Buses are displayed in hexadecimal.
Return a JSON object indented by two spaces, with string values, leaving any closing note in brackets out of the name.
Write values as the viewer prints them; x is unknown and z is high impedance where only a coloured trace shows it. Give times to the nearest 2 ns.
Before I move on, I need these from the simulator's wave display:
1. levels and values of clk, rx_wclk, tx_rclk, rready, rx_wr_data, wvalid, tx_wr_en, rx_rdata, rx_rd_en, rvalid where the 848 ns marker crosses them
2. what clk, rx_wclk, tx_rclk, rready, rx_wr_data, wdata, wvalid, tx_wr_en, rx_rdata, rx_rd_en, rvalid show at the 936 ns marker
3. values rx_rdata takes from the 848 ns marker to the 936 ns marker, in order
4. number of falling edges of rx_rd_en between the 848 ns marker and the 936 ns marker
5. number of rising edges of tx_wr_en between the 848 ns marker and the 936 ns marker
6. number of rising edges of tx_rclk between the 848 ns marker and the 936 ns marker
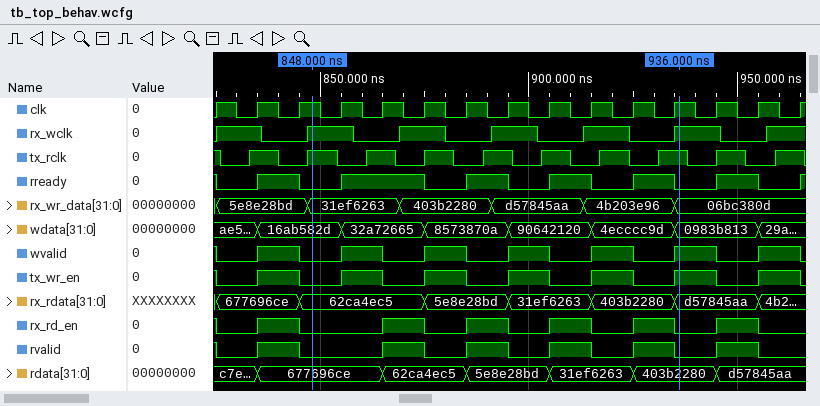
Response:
{
  "levels and values of clk, rx_wclk, tx_rclk, rready, rx_wr_data, wvalid, tx_wr_en, rx_rdata, rx_rd_en, rvalid where the 848 ns marker crosses them": "clk=1, rx_wclk=1, tx_rclk=1, rready=0, rx_wr_data=31ef6263, wvalid=0, tx_wr_en=0, rx_rdata=62ca4ec5, rx_rd_en=0, rvalid=0",
  "what clk, rx_wclk, tx_rclk, rready, rx_wr_data, wdata, wvalid, tx_wr_en, rx_rdata, rx_rd_en, rvalid show at the 936 ns marker": "clk=1, rx_wclk=1, tx_rclk=1, rready=0, rx_wr_data=06bc380d, wdata=0983b813, wvalid=1, tx_wr_en=1, rx_rdata=d57845aa, rx_rd_en=0, rvalid=0",
  "values rx_rdata takes from the 848 ns marker to the 936 ns marker, in order": "62ca4ec5, 5e8e28bd, 31ef6263, 403b2280, d57845aa",
  "number of falling edges of rx_rd_en between the 848 ns marker and the 936 ns marker": "4",
  "number of rising edges of tx_wr_en between the 848 ns marker and the 936 ns marker": "5",
  "number of rising edges of tx_rclk between the 848 ns marker and the 936 ns marker": "6"
}
